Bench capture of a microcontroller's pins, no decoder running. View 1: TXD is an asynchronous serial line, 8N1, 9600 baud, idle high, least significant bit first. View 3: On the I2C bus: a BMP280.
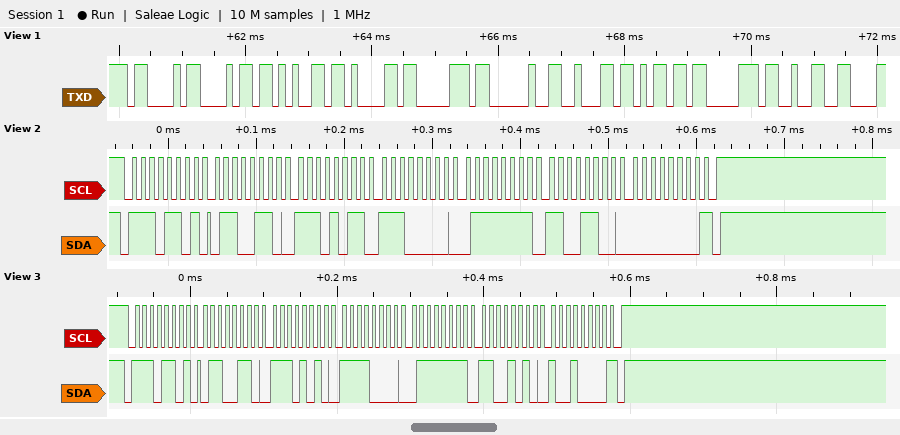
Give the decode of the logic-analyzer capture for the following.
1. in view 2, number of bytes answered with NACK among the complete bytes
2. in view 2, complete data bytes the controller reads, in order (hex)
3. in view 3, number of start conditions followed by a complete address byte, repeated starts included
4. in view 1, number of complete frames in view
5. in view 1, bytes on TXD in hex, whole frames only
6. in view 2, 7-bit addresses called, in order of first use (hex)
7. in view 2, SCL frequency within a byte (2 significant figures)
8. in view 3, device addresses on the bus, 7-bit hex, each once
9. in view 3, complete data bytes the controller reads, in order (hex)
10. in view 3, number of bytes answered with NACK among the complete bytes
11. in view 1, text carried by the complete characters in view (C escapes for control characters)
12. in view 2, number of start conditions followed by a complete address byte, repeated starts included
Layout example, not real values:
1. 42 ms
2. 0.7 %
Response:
1. 1
2. 66 EB E0 7F CC 00
3. 1
4. 10
5. 0x43 0x68 0x65 0x61 0x70 0x20 0x62 0x6D 0x70 0x32
6. 0x76
7. 100 kHz
8. 0x76
9. 66 EA F0 7F CA 90
10. 1
11. "Cheap bmp2"
12. 1
